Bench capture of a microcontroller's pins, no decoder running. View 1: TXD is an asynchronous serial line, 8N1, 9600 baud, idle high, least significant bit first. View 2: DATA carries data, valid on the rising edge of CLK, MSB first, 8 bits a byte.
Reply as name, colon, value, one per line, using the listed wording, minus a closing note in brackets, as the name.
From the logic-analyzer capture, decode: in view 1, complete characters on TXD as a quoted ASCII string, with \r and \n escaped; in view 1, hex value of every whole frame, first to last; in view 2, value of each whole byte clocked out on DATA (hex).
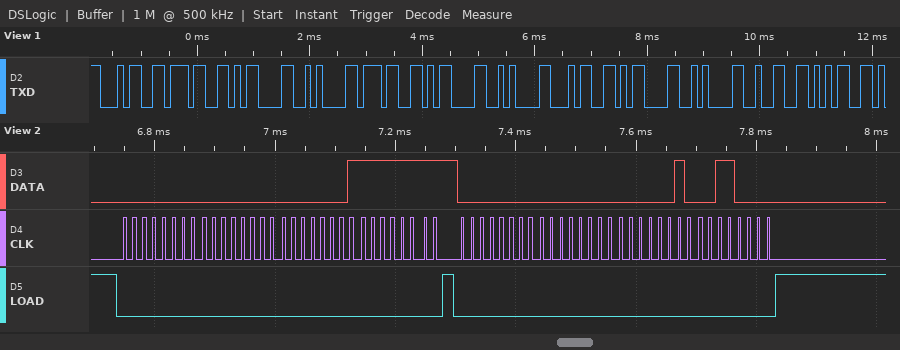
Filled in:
in view 1, complete characters on TXD as a quoted ASCII string, with \r and \n escaped: "47\r\n7\r\n4\r\n25"
in view 1, hex value of every whole frame, first to last: 34 37 0D 0A 37 0D 0A 34 0D 0A 32 35
in view 2, value of each whole byte clocked out on DATA: 00 00 01 FF 00 00 02 30
